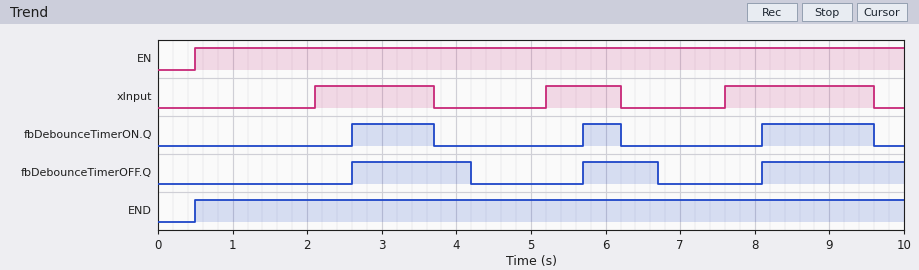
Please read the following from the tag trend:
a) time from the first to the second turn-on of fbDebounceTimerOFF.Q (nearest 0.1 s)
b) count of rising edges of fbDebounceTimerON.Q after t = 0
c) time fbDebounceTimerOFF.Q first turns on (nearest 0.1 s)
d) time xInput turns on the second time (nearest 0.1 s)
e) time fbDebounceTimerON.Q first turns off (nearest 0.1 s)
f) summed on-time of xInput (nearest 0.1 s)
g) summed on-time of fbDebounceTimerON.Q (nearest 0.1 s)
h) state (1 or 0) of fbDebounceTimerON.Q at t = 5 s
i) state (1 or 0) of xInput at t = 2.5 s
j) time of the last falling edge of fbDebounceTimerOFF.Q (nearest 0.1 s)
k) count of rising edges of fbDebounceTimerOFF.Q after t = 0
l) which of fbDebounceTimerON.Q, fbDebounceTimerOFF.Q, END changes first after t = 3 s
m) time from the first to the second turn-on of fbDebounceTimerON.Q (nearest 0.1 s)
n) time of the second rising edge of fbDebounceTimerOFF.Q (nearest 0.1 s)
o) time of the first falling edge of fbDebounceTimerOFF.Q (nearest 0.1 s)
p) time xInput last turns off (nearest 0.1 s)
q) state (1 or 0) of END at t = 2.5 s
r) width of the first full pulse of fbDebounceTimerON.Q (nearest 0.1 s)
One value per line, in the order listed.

3.1 s
3
2.6 s
5.2 s
3.7 s
4.6 s
3.1 s
0
1
6.7 s
3
fbDebounceTimerON.Q
3.1 s
5.7 s
4.2 s
9.6 s
1
1.1 s
